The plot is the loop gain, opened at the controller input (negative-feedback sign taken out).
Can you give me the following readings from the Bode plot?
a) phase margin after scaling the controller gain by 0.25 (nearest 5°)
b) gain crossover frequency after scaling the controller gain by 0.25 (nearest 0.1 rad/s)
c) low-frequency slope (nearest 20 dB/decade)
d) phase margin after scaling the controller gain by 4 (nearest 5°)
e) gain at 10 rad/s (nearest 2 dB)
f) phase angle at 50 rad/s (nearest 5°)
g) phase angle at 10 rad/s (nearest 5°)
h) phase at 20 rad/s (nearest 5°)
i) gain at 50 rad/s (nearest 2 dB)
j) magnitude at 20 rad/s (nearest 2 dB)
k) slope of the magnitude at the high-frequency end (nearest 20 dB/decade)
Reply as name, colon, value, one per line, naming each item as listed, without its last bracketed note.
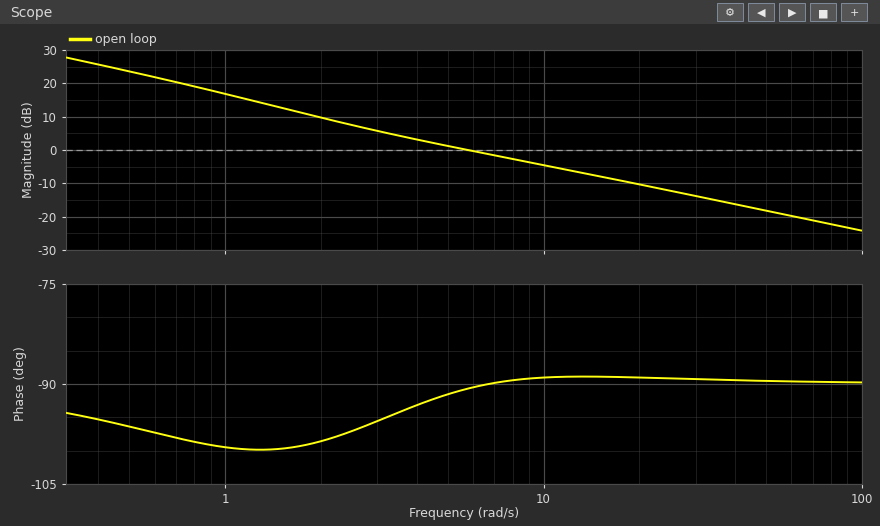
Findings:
phase margin after scaling the controller gain by 0.25: 80°
gain crossover frequency after scaling the controller gain by 0.25: 1.6 rad/s
low-frequency slope: -20 dB/decade
phase margin after scaling the controller gain by 4: 90°
gain at 10 rad/s: -4 dB
phase angle at 50 rad/s: -90°
phase angle at 10 rad/s: -90°
phase at 20 rad/s: -90°
gain at 50 rad/s: -18 dB
magnitude at 20 rad/s: -10 dB
slope of the magnitude at the high-frequency end: -20 dB/decade
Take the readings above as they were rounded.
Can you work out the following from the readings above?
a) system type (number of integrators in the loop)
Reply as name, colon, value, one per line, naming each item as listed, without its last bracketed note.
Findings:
system type: 1
